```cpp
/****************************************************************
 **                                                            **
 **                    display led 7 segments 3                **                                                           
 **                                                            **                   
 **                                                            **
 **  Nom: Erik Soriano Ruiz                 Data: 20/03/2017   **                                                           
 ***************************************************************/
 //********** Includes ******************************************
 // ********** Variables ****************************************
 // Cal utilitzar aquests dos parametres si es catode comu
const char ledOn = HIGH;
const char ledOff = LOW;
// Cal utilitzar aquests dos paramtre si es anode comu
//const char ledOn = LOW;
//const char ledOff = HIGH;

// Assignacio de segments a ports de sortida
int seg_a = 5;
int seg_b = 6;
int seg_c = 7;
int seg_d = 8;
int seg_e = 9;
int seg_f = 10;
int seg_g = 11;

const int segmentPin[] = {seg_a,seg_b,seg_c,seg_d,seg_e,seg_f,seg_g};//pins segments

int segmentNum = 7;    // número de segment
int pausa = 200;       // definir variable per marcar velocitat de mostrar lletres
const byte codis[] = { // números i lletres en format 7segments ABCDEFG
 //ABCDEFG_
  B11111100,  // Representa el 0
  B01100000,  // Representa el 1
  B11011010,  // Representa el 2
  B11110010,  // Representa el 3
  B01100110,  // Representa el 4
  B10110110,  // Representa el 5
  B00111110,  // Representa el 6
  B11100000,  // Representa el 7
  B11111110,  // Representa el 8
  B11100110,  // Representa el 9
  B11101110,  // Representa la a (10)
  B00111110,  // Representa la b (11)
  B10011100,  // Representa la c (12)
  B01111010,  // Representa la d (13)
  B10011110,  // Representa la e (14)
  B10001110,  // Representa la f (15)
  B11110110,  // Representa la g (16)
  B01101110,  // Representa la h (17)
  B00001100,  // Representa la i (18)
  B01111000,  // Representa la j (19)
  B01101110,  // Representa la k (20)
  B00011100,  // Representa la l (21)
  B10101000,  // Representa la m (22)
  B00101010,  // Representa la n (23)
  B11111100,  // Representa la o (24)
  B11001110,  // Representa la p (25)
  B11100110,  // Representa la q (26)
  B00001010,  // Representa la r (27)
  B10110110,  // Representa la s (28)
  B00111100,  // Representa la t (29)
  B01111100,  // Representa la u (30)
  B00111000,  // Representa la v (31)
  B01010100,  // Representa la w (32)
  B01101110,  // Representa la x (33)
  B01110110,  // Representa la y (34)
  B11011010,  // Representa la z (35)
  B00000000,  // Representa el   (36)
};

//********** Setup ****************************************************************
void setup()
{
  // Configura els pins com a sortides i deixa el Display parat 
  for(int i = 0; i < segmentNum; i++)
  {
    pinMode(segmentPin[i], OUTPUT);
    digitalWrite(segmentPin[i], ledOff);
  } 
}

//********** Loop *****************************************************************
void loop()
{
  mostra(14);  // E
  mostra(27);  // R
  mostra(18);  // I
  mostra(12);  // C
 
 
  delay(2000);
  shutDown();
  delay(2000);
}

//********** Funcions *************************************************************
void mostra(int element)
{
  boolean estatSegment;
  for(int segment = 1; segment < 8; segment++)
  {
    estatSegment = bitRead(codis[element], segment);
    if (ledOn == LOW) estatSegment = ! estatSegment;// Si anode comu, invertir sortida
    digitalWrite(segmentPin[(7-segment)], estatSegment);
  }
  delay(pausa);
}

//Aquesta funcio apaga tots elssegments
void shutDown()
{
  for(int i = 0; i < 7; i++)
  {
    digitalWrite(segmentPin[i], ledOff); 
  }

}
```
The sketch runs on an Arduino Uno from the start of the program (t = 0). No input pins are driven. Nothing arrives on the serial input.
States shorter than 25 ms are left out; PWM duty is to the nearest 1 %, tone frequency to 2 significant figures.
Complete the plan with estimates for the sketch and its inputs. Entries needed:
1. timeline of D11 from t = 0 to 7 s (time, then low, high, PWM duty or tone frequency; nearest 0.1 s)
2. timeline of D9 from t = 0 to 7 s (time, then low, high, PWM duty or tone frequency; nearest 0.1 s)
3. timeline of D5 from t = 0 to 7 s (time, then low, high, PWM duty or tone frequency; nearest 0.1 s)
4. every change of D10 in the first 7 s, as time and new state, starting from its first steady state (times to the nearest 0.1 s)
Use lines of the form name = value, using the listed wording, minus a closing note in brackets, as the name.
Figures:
timeline of D11 from t = 0 to 7 s = 0 s high; 0.4 s low; 4.8 s high; 5.2 s low
timeline of D9 from t = 0 to 7 s = 0 s high; 2.8 s low; 4.8 s high
timeline of D5 from t = 0 to 7 s = 0 s high; 0.2 s low; 0.6 s high; 2.8 s low; 4.8 s high; 5 s low; 5.4 s high
every change of D10 in the first 7 s, as time and new state, starting from its first steady state = 0 s high; 0.2 s low; 0.4 s high; 2.8 s low; 4.8 s high; 5 s low; 5.2 s high
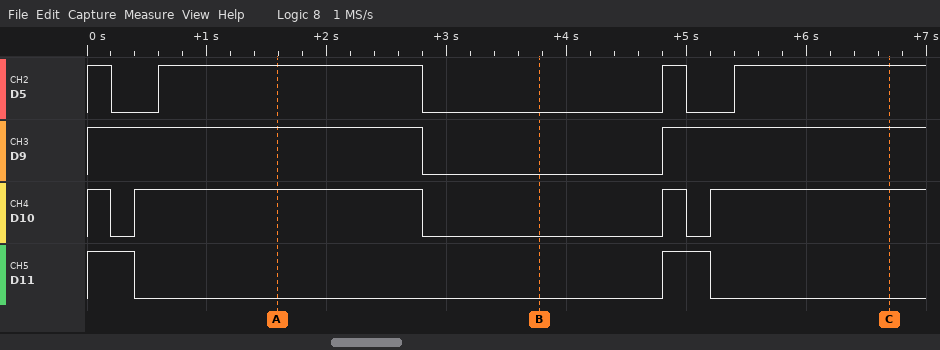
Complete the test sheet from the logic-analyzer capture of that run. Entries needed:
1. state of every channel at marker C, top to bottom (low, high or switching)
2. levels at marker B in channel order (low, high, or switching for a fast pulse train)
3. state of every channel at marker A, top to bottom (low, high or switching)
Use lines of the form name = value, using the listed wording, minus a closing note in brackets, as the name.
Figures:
state of every channel at marker C, top to bottom = D5 high, D9 high, D10 high, D11 low
levels at marker B in channel order = D5 low, D9 low, D10 low, D11 low
state of every channel at marker A, top to bottom = D5 high, D9 high, D10 high, D11 low
